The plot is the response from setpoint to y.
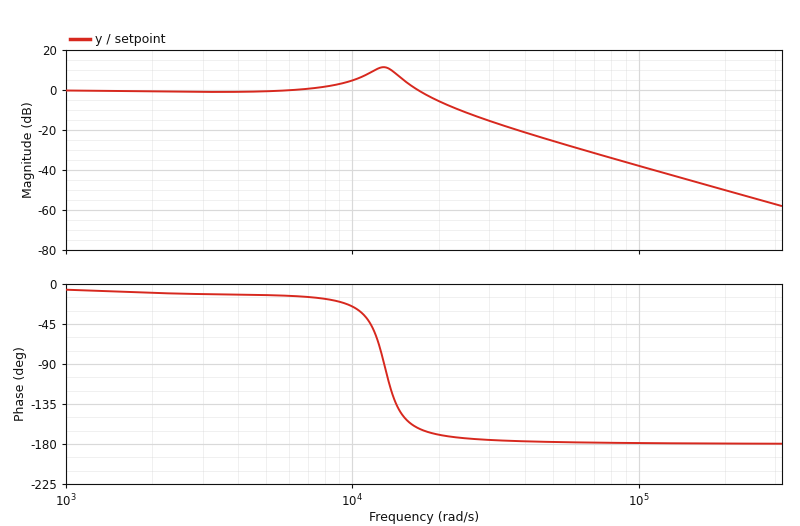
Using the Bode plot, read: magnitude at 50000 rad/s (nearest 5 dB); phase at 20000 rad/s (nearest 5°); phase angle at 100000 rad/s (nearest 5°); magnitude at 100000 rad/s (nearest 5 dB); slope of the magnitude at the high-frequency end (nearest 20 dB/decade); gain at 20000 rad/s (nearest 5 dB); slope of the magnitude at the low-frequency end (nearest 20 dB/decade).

-25 dB
-170°
-180°
-40 dB
-40 dB/decade
-5 dB
0 dB/decade
